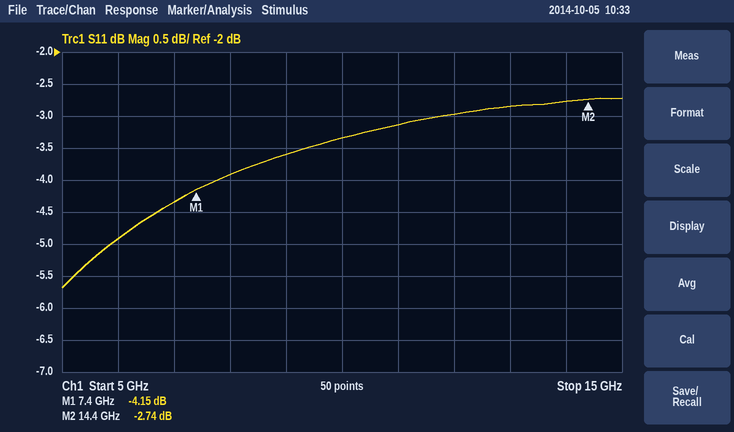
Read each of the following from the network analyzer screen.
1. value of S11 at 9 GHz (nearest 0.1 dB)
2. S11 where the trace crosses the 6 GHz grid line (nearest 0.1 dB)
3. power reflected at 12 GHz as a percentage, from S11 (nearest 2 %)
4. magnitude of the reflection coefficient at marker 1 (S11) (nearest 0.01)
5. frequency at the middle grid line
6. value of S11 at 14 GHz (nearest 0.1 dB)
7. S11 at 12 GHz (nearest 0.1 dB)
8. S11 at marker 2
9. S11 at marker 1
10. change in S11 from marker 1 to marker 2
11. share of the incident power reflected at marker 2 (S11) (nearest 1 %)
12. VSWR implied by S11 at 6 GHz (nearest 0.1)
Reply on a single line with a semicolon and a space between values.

-3.6 dB; -4.9 dB; 50 %; 0.62; 10 GHz; -2.8 dB; -3.0 dB; -2.74 dB; -4.15 dB; 1.41 dB; 53 %; 3.6
